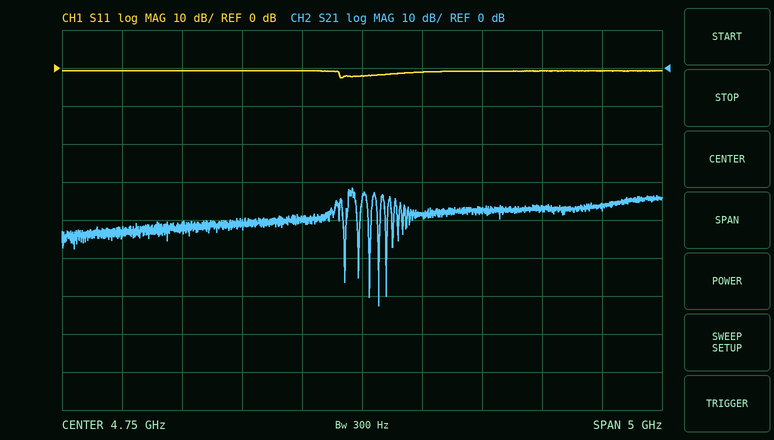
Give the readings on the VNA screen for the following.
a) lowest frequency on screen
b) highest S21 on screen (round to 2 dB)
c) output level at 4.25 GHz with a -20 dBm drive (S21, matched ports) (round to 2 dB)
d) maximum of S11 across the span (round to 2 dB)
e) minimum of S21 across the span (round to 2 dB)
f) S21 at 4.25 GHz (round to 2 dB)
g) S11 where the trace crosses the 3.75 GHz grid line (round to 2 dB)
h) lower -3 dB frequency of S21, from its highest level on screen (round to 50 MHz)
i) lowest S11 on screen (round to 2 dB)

2.25 GHz
-32 dB
-60 dBm
0 dB
-62 dB
-40 dB
0 dB
4.65 GHz
-2 dB
